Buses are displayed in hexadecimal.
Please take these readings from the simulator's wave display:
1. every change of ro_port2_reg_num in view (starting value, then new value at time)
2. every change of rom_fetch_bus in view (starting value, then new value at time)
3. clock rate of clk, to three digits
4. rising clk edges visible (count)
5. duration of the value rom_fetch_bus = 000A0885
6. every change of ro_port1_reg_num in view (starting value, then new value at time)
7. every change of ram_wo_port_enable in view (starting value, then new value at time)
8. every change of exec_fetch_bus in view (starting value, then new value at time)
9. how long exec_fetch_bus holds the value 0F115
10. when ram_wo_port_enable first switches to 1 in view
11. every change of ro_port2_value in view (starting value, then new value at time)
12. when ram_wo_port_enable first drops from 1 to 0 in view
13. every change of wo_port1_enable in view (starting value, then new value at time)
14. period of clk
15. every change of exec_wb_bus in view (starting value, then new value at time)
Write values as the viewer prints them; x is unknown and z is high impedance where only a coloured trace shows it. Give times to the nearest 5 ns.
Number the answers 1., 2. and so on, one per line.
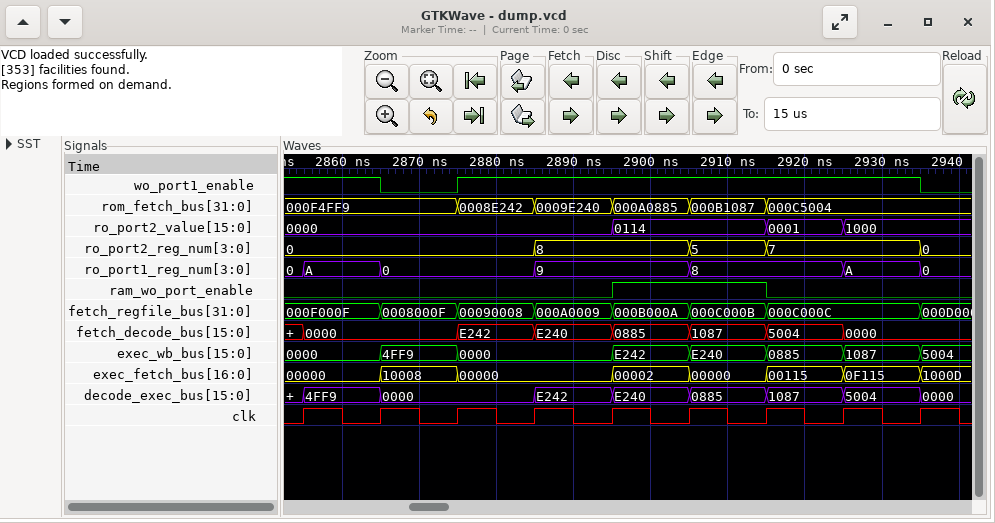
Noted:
1. 0, 8 at 2885 ns, 5 at 2905 ns, 7 at 2915 ns, 0 at 2935 ns
2. 000F4FF9, 0008E242 at 2875 ns, 0009E240 at 2885 ns, 000A0885 at 2895 ns, 000B1087 at 2905 ns, 000C5004 at 2915 ns
3. 100 MHz
4. 9
5. 10 ns
6. 0, A at 2855 ns, 0 at 2865 ns, 9 at 2885 ns, 8 at 2905 ns, A at 2925 ns, 0 at 2935 ns
7. 0, 1 at 2895 ns, 0 at 2915 ns
8. 00000, 10008 at 2865 ns, 00000 at 2875 ns, 00002 at 2895 ns, 00000 at 2905 ns, 00115 at 2915 ns, 0F115 at 2925 ns, 1000D at 2935 ns
9. 10 ns
10. 2895 ns
11. 0000, 0114 at 2895 ns, 0001 at 2915 ns, 1000 at 2925 ns
12. 2915 ns
13. 1, 0 at 2865 ns, 1 at 2875 ns, 0 at 2935 ns
14. 10 ns
15. 0000, 4FF9 at 2865 ns, 0000 at 2875 ns, E242 at 2895 ns, E240 at 2905 ns, 0885 at 2915 ns, 1087 at 2925 ns, 5004 at 2935 ns
